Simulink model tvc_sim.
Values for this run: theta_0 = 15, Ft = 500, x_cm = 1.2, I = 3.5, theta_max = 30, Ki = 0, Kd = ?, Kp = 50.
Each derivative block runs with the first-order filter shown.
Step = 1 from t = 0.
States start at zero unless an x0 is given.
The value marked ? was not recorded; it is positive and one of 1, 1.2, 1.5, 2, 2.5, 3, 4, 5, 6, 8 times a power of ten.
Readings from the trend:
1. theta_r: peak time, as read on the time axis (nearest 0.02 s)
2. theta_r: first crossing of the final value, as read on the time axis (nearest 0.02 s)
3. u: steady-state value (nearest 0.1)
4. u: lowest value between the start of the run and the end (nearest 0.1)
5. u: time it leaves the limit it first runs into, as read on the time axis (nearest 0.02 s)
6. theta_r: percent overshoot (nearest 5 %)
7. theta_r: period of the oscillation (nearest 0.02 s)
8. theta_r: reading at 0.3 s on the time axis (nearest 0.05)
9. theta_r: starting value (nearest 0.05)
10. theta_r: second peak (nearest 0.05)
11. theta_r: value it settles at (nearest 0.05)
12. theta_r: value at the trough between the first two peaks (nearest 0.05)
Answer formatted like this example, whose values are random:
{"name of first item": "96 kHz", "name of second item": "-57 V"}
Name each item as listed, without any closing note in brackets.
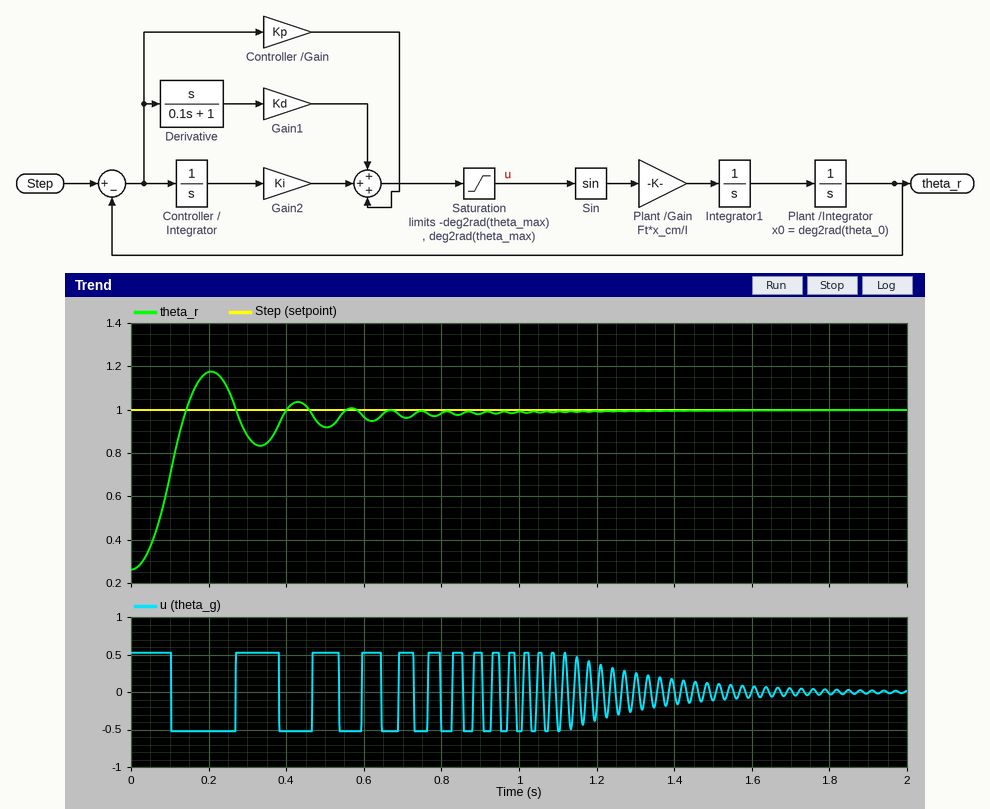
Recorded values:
{"theta_r: peak time, as read on the time axis": "0.20 s", "theta_r: first crossing of the final value, as read on the time axis": "0.14 s", "u: steady-state value": "0.0", "u: lowest value between the start of the run and the end": "-0.5", "u: time it leaves the limit it first runs into, as read on the time axis": "0.10 s", "theta_r: percent overshoot": "25 %", "theta_r: period of the oscillation": "0.22 s", "theta_r: reading at 0.3 s on the time axis": "0.90", "theta_r: starting value": "0.25", "theta_r: second peak": "1.05", "theta_r: value it settles at": "1.00", "theta_r: value at the trough between the first two peaks": "0.85"}
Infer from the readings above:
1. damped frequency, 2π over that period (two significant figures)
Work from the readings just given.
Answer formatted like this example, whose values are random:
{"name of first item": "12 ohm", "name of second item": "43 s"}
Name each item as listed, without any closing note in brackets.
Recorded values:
{"damped frequency, 2π over that period": "29 rad/s"}
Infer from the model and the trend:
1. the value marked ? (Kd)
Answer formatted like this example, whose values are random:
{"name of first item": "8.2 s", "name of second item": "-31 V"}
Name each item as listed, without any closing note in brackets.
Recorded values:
{"the value marked ?": "20"}
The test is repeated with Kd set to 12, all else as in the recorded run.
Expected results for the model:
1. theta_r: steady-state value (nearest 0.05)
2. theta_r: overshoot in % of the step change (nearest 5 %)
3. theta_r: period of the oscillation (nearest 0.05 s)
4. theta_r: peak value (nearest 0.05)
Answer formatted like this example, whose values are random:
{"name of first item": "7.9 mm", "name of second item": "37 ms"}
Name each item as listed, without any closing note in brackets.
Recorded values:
{"theta_r: steady-state value": "1.00", "theta_r: overshoot in % of the step change": "35 %", "theta_r: period of the oscillation": "0.25 s", "theta_r: peak value": "1.25"}
